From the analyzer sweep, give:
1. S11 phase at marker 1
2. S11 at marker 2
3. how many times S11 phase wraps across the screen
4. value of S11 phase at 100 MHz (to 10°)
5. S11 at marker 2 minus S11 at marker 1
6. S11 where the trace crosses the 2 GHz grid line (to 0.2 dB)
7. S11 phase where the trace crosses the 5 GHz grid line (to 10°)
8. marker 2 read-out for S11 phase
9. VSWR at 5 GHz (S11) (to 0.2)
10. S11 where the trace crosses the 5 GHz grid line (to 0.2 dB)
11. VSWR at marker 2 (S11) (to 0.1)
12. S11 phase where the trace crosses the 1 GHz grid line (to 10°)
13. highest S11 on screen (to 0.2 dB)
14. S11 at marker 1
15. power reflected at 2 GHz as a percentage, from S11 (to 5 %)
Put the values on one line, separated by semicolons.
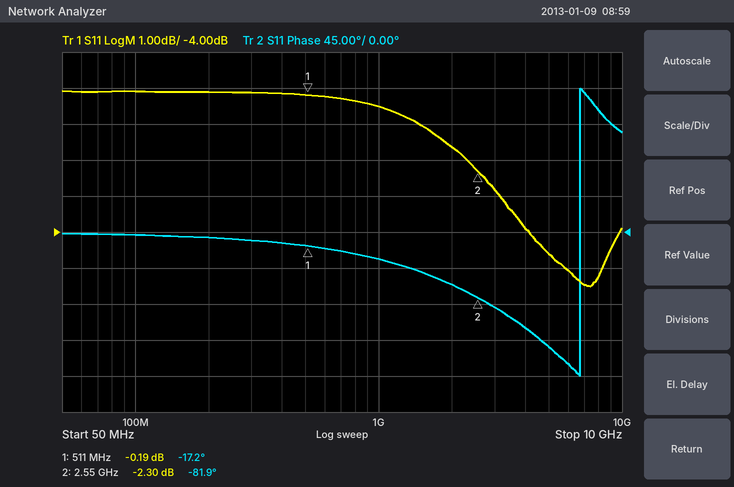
-17.2°; -2.30 dB; 1; 0°; -2.11 dB; -1.6 dB; -140°; -81.9°; 3.8; -4.6 dB; 7.6; -30°; 0.0 dB; -0.19 dB; 70 %
